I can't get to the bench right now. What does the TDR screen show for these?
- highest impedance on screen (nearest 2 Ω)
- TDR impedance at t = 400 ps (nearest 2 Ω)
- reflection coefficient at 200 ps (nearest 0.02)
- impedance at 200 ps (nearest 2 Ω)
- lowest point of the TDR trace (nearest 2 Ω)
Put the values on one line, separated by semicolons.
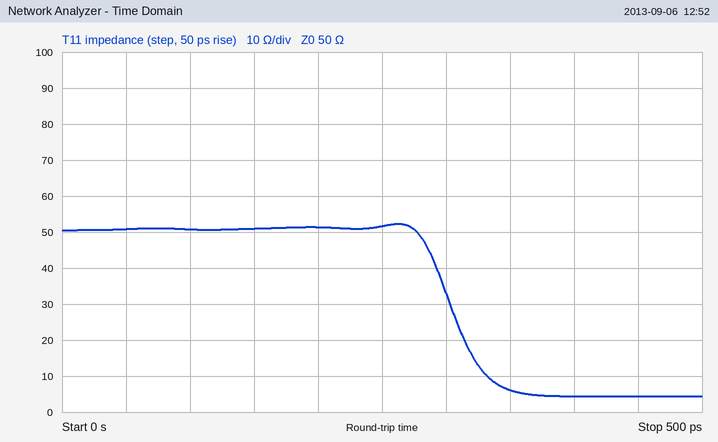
52 Ω; 4 Ω; +0.02; 52 Ω; 4 Ω
